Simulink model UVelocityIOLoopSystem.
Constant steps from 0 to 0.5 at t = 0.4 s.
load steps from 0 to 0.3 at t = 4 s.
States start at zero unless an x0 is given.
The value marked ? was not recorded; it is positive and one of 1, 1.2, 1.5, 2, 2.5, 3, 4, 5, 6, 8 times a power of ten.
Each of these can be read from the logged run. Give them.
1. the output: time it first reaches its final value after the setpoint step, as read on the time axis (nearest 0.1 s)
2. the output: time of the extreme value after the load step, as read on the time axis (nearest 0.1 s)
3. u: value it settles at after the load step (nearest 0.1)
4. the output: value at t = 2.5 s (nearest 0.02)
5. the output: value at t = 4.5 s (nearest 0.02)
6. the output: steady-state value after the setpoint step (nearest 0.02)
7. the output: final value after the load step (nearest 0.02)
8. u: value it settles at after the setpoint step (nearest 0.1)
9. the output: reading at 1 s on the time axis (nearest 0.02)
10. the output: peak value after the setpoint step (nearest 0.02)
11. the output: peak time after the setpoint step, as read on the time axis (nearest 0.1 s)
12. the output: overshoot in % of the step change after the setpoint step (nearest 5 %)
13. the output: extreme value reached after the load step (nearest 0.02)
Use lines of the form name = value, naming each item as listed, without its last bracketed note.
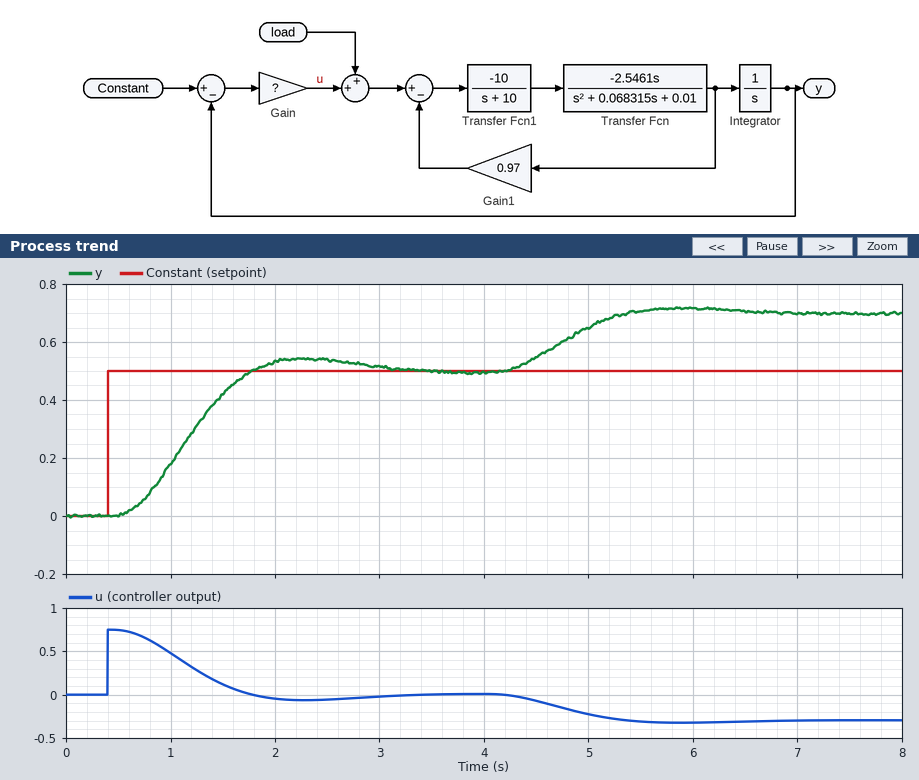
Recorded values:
the output: time it first reaches its final value after the setpoint step, as read on the time axis = 1.8 s
the output: time of the extreme value after the load step, as read on the time axis = 5.9 s
u: value it settles at after the load step = -0.3
the output: value at t = 2.5 s = 0.54
the output: value at t = 4.5 s = 0.54
the output: steady-state value after the setpoint step = 0.50
the output: final value after the load step = 0.70
u: value it settles at after the setpoint step = 0.0
the output: reading at 1 s on the time axis = 0.18
the output: peak value after the setpoint step = 0.54
the output: peak time after the setpoint step, as read on the time axis = 2.3 s
the output: overshoot in % of the step change after the setpoint step = 10 %
the output: extreme value reached after the load step = 0.72
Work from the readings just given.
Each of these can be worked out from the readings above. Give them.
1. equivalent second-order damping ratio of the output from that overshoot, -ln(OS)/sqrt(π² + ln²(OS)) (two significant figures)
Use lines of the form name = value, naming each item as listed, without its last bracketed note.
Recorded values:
equivalent second-order damping ratio of the output from that overshoot, -ln(OS)/sqrt(π² + ln²(OS)) = 0.59
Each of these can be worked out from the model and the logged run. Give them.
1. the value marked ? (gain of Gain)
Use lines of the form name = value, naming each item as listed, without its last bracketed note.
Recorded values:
the value marked ? = 1.5
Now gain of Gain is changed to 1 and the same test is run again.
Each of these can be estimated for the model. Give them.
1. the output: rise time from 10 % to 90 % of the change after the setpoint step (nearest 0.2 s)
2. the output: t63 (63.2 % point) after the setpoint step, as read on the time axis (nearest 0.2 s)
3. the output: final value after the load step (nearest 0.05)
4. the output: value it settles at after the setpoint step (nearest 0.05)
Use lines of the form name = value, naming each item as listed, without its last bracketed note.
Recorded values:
the output: rise time from 10 % to 90 % of the change after the setpoint step = 1.4 s
the output: t63 (63.2 % point) after the setpoint step, as read on the time axis = 1.6 s
the output: final value after the load step = 0.80
the output: value it settles at after the setpoint step = 0.50
